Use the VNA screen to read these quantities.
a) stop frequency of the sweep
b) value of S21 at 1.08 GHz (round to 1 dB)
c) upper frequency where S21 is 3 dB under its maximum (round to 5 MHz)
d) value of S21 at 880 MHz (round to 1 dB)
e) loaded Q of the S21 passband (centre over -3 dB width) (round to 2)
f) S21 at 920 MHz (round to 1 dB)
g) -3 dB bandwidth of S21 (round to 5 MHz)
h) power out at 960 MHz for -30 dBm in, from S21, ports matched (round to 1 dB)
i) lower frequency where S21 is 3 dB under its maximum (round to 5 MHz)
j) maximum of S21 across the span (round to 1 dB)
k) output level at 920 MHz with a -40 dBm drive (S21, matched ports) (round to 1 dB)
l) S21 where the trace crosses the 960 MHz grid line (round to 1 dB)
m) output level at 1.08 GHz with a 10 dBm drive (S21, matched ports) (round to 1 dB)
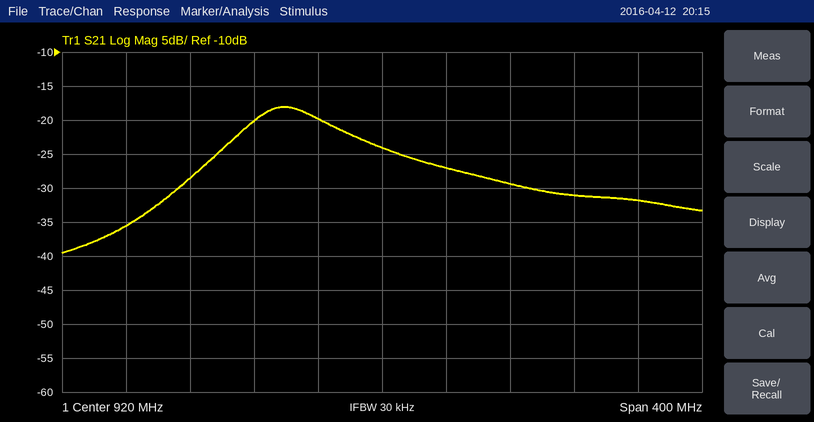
1.12 GHz
-32 dB
890 MHz
-20 dB
16
-24 dB
55 MHz
-57 dBm
835 MHz
-18 dB
-64 dBm
-27 dB
-22 dBm
